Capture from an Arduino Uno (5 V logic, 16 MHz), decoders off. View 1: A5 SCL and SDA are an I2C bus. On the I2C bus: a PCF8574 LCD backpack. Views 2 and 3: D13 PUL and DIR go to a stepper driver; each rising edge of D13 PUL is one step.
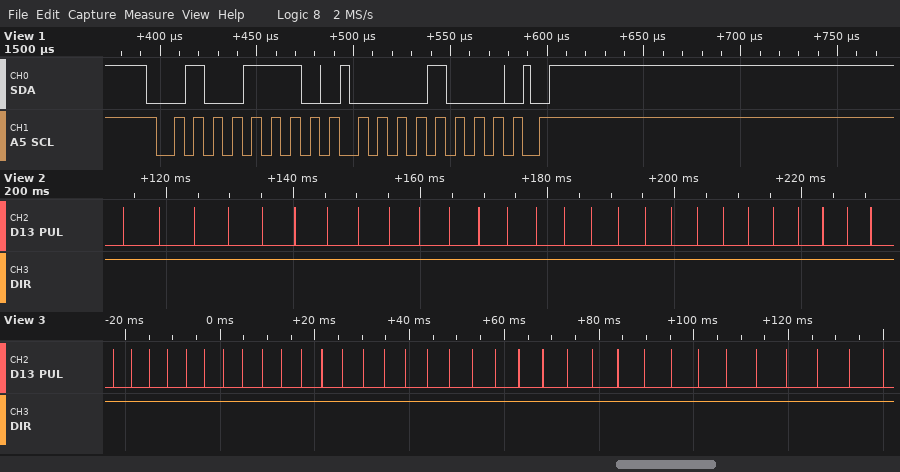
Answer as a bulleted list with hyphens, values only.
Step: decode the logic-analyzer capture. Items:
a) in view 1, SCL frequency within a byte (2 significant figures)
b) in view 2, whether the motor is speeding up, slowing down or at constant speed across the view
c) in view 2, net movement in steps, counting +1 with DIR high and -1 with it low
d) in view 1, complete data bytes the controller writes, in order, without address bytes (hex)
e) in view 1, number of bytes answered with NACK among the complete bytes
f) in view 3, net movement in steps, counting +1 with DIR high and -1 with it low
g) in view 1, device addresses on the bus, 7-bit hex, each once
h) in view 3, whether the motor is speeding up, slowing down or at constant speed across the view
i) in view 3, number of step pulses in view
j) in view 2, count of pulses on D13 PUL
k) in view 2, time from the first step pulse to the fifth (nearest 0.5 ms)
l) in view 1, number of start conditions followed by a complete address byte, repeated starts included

- 100 kHz
- speeding up
- +27
- 08
- 0
- +34
- 0x27
- slowing down
- 34
- 27
- 22.0 ms
- 1
